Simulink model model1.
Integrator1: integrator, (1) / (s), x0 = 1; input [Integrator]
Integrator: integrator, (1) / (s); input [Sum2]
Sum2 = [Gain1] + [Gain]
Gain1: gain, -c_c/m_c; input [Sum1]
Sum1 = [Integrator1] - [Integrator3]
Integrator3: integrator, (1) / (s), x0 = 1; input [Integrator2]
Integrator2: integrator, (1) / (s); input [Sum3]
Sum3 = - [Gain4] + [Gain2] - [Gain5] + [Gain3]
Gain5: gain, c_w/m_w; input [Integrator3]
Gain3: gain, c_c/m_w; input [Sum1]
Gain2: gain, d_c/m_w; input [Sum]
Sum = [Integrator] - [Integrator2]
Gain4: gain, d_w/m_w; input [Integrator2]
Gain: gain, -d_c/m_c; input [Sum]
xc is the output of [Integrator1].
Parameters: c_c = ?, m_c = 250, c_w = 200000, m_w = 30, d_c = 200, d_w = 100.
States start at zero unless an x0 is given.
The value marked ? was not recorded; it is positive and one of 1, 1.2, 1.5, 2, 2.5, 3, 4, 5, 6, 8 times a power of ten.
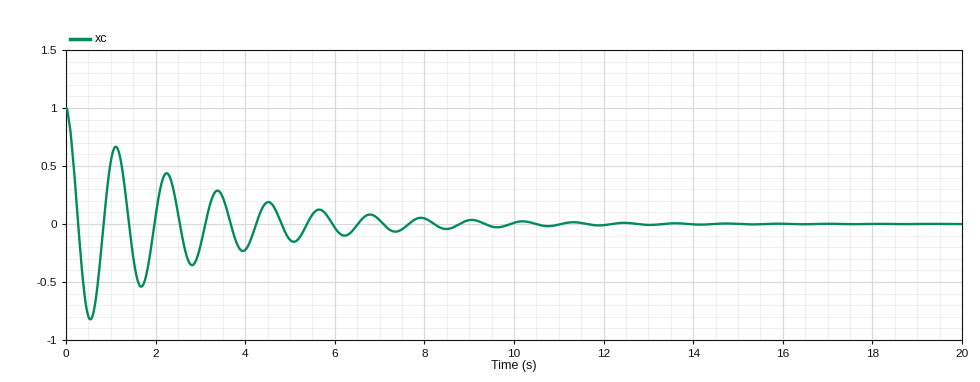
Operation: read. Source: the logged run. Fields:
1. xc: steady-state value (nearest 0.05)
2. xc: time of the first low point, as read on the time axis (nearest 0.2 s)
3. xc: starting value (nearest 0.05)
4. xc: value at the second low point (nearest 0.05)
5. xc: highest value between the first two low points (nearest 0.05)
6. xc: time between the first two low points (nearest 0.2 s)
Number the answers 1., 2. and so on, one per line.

1. 0.00
2. 0.6 s
3. 1.00
4. -0.55
5. 0.65
6. 1.2 s
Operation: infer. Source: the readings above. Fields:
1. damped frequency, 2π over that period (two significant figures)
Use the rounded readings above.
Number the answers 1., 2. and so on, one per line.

1. 5.2 rad/s
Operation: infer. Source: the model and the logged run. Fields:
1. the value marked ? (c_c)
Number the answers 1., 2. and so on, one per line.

1. 8000
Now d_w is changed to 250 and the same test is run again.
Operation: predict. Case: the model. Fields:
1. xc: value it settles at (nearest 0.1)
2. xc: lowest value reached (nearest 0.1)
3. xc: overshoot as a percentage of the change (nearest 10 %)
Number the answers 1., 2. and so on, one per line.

1. 0.0
2. -0.8
3. 80 %
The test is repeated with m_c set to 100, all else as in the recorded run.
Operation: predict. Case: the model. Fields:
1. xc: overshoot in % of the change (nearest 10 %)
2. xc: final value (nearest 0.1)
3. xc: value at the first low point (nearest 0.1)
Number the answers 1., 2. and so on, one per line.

1. 70 %
2. 0.0
3. -0.7
